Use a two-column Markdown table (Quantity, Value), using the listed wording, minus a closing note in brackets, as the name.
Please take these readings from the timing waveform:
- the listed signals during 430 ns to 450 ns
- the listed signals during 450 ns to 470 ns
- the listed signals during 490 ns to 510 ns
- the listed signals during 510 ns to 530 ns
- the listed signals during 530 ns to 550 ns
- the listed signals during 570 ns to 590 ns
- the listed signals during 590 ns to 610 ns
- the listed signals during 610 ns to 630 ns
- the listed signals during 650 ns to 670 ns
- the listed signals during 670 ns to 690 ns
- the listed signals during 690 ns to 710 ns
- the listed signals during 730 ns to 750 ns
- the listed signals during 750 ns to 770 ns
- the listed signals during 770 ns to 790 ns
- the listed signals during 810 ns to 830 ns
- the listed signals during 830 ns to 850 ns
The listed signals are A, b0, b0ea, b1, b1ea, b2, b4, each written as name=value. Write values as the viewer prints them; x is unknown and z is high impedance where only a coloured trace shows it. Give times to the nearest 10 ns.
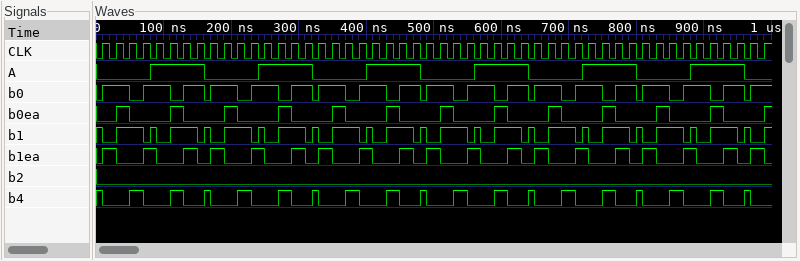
| Quantity | Value |
|---|---|
| the listed signals during 430 ns to 450 ns | A=1, b0=0, b0ea=1, b1=1, b1ea=0, b2=0, b4=1 |
| the listed signals during 450 ns to 470 ns | A=1, b0=1, b0ea=0, b1=1, b1ea=1, b2=0, b4=0 |
| the listed signals during 490 ns to 510 ns | A=0, b0=1, b0ea=0, b1=0, b1ea=1, b2=0, b4=0 |
| the listed signals during 510 ns to 530 ns | A=0, b0=1, b0ea=1, b1=1, b1ea=0, b2=0, b4=0 |
| the listed signals during 530 ns to 550 ns | A=0, b0=0, b0ea=0, b1=1, b1ea=0, b2=0, b4=1 |
| the listed signals during 570 ns to 590 ns | A=1, b0=1, b0ea=0, b1=0, b1ea=0, b2=0, b4=0 |
| the listed signals during 590 ns to 610 ns | A=1, b0=0, b0ea=1, b1=1, b1ea=0, b2=0, b4=1 |
| the listed signals during 610 ns to 630 ns | A=1, b0=1, b0ea=0, b1=1, b1ea=1, b2=0, b4=0 |
| the listed signals during 650 ns to 670 ns | A=0, b0=1, b0ea=0, b1=0, b1ea=1, b2=0, b4=0 |
| the listed signals during 670 ns to 690 ns | A=0, b0=1, b0ea=1, b1=1, b1ea=0, b2=0, b4=0 |
| the listed signals during 690 ns to 710 ns | A=0, b0=0, b0ea=0, b1=1, b1ea=0, b2=0, b4=1 |
| the listed signals during 730 ns to 750 ns | A=1, b0=1, b0ea=0, b1=0, b1ea=0, b2=0, b4=0 |
| the listed signals during 750 ns to 770 ns | A=1, b0=0, b0ea=1, b1=1, b1ea=0, b2=0, b4=1 |
| the listed signals during 770 ns to 790 ns | A=1, b0=1, b0ea=0, b1=1, b1ea=1, b2=0, b4=0 |
| the listed signals during 810 ns to 830 ns | A=0, b0=1, b0ea=0, b1=0, b1ea=1, b2=0, b4=0 |
| the listed signals during 830 ns to 850 ns | A=0, b0=1, b0ea=1, b1=1, b1ea=0, b2=0, b4=0 |
